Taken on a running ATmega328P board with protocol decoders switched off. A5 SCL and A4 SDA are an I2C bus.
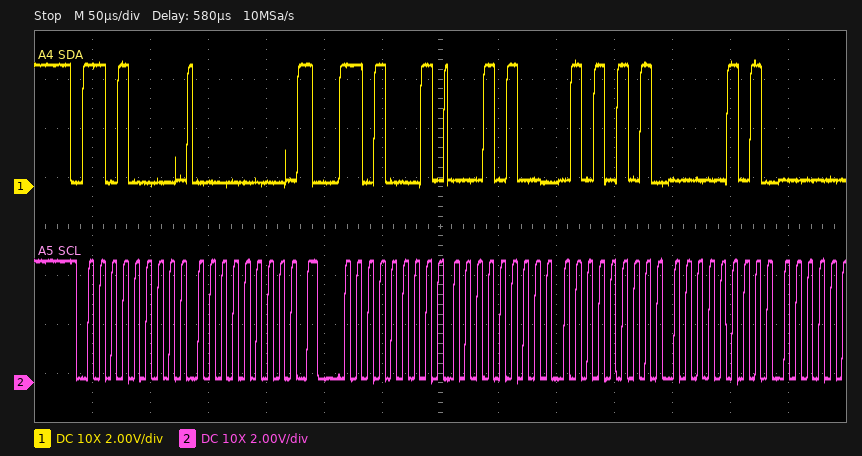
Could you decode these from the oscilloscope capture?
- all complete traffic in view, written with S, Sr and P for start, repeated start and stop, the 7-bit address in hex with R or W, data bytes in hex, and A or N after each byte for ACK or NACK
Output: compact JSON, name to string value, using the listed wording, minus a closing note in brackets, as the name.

{"all complete traffic in view, written with S, Sr and P for start, repeated start and stop, the 7-bit address in hex with R or W, data bytes in hex, and A or N after each byte for ACK or NACK": "S 68W A 00 A Sr 68R A 14 A 55 A 05 A"}
